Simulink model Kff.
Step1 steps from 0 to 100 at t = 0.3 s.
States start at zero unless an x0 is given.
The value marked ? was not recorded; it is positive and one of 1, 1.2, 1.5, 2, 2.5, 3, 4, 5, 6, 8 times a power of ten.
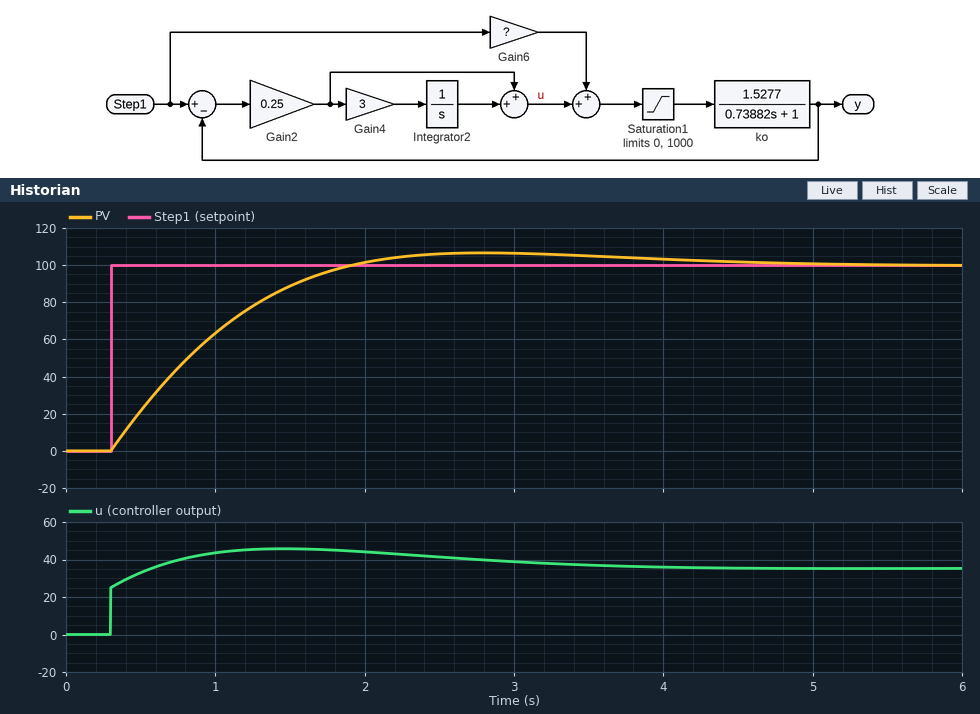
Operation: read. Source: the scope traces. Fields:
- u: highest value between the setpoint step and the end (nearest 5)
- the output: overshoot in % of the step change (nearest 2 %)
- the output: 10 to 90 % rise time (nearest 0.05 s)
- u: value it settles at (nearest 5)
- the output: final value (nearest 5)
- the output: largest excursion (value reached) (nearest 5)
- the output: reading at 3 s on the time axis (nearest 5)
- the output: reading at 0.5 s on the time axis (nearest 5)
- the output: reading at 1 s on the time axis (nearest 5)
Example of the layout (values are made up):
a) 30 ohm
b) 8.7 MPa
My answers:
a) 45
b) 6 %
c) 1.15 s
d) 35
e) 100
f) 105
g) 105
h) 20
i) 65
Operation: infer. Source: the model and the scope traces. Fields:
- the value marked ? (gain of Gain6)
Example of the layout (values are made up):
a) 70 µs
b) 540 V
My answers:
a) 0.3
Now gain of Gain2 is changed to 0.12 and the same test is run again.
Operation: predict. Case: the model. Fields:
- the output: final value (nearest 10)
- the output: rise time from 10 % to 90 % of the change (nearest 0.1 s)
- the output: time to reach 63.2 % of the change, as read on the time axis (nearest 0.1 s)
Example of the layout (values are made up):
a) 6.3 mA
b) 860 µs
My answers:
a) 100
b) 2.1 s
c) 1.4 s
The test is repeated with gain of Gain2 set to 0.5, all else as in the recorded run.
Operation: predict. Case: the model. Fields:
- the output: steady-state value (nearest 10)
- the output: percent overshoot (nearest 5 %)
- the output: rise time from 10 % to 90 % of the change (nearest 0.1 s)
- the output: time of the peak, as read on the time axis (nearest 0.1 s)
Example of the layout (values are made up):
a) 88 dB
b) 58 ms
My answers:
a) 100
b) 10 %
c) 0.7 s
d) 1.9 s
